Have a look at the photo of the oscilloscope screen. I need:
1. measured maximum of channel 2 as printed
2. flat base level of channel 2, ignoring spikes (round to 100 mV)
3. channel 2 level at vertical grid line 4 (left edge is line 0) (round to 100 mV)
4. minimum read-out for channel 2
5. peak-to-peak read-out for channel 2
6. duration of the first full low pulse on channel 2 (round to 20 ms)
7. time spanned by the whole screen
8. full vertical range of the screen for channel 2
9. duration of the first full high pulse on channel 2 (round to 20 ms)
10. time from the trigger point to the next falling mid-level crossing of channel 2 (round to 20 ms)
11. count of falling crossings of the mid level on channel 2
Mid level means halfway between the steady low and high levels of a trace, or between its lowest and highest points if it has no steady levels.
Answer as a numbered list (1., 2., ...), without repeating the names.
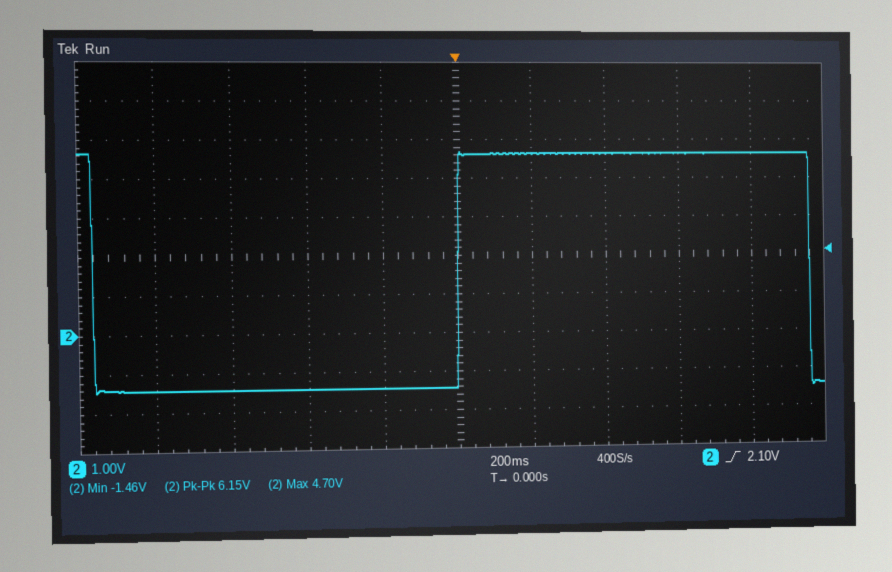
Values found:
1. 4.70 V
2. -1.4 V
3. -1.4 V
4. -1.46 V
5. 6.15 V
6. 960 ms
7. 2 s
8. 10 V
9. 960 ms
10. 960 ms
11. 2
